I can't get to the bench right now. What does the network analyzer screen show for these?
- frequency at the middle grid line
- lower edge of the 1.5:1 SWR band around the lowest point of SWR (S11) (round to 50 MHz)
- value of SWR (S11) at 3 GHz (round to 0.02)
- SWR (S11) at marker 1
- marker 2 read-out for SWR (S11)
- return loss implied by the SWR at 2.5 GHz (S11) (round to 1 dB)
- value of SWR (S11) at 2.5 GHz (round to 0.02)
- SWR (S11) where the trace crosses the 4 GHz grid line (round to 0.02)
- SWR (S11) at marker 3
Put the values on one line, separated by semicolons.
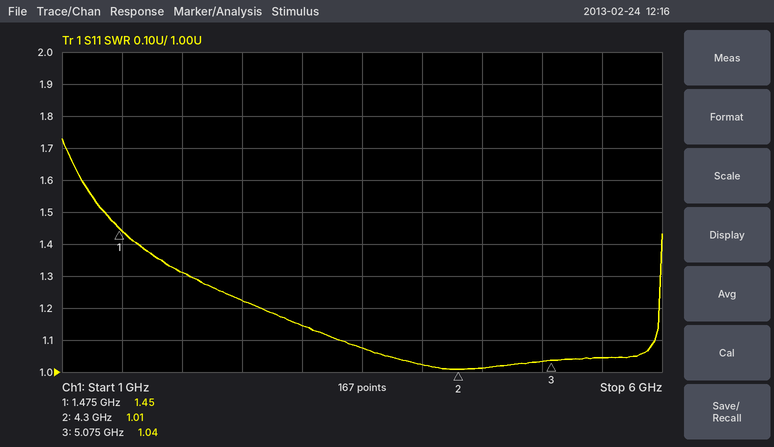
3.5 GHz; 1.35 GHz; 1.14; 1.45; 1.01; 20 dB; 1.22; 1.02; 1.04
